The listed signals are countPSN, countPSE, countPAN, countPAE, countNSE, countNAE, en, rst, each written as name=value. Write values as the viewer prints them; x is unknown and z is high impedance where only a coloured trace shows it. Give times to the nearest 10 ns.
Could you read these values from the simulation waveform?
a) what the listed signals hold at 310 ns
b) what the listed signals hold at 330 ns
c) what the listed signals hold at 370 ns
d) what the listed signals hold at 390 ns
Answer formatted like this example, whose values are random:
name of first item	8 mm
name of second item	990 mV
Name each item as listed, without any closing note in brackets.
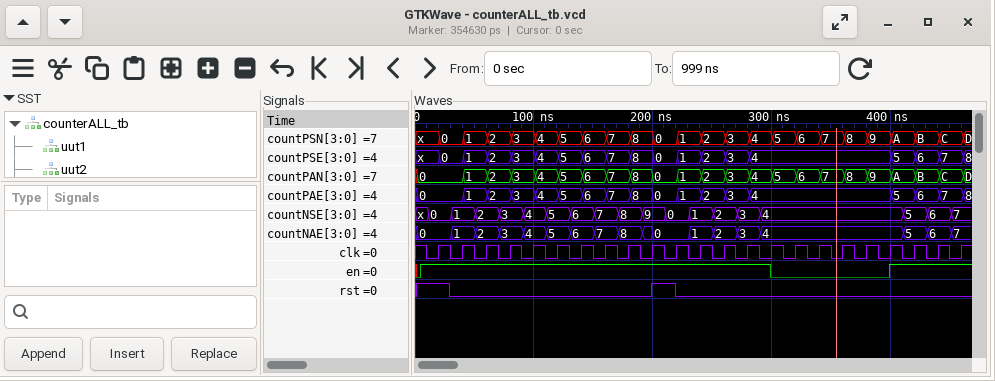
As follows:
what the listed signals hold at 310 ns	countPSN=5, countPSE=4, countPAN=5, countPAE=4, countNSE=4, countNAE=4, en=0, rst=0
what the listed signals hold at 330 ns	countPSN=6, countPSE=4, countPAN=6, countPAE=4, countNSE=4, countNAE=4, en=0, rst=0
what the listed signals hold at 370 ns	countPSN=8, countPSE=4, countPAN=8, countPAE=4, countNSE=4, countNAE=4, en=0, rst=0
what the listed signals hold at 390 ns	countPSN=9, countPSE=4, countPAN=9, countPAE=4, countNSE=4, countNAE=4, en=0, rst=0
